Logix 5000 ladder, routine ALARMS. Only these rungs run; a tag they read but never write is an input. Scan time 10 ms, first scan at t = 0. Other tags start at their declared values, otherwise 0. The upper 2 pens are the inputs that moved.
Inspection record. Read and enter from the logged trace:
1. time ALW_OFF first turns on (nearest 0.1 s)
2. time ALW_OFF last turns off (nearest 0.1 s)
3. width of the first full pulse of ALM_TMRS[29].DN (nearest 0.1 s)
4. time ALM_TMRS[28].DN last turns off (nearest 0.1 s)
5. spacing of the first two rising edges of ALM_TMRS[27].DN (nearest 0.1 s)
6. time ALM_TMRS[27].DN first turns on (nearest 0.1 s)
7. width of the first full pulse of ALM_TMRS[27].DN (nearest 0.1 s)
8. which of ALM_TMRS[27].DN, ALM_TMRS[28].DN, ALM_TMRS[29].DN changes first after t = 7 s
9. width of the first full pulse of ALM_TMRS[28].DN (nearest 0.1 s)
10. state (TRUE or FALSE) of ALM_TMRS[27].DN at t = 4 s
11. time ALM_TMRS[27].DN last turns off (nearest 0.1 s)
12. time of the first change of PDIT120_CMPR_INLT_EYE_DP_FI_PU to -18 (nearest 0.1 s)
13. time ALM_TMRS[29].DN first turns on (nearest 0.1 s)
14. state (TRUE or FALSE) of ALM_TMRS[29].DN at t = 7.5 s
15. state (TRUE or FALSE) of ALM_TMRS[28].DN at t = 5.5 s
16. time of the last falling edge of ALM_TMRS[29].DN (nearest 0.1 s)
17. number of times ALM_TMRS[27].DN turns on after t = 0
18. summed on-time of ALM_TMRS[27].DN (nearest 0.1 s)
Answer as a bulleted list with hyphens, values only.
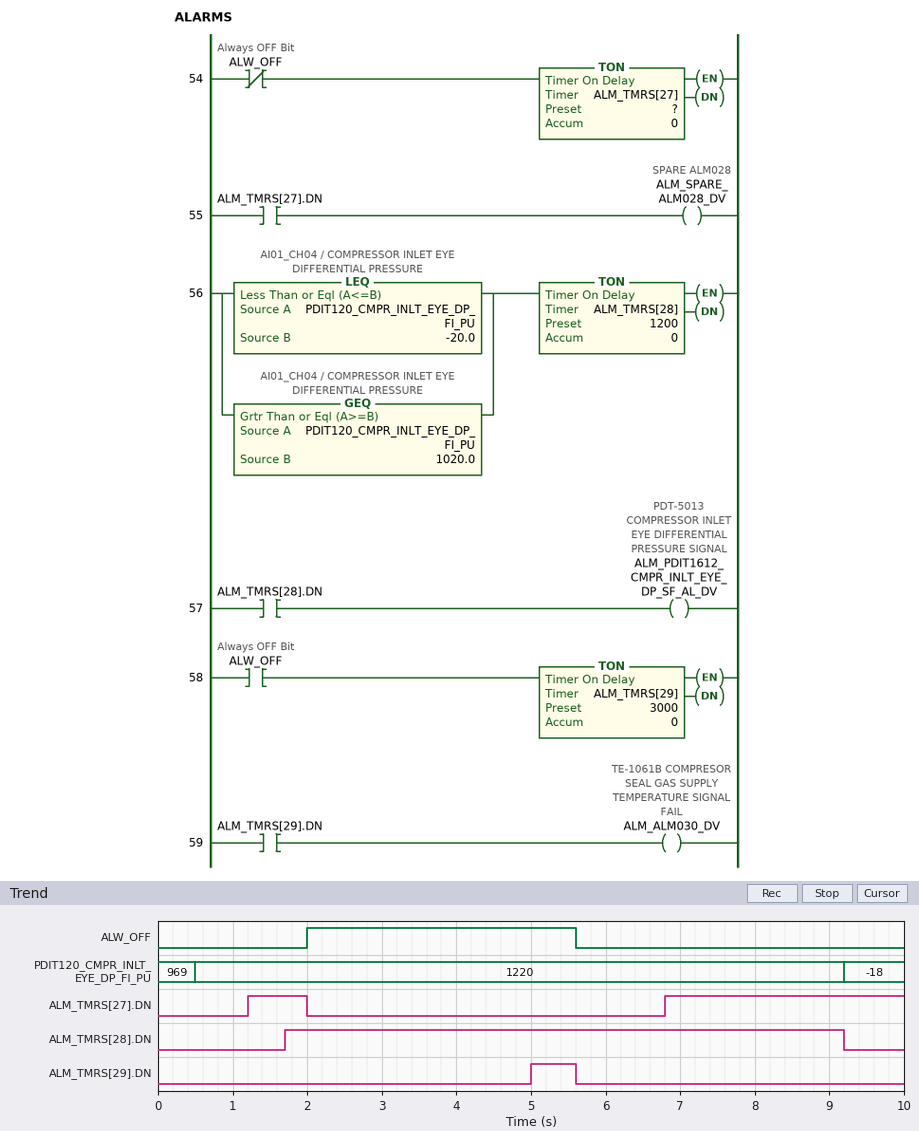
- 2.0 s
- 5.6 s
- 0.6 s
- 9.2 s
- 5.6 s
- 1.2 s
- 0.8 s
- ALM_TMRS[28].DN
- 7.5 s
- FALSE
- 2.0 s
- 9.2 s
- 5.0 s
- FALSE
- TRUE
- 5.6 s
- 2
- 4.0 s
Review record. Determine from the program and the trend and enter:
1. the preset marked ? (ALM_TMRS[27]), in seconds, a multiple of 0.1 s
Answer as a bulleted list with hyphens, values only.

- 1.2 s
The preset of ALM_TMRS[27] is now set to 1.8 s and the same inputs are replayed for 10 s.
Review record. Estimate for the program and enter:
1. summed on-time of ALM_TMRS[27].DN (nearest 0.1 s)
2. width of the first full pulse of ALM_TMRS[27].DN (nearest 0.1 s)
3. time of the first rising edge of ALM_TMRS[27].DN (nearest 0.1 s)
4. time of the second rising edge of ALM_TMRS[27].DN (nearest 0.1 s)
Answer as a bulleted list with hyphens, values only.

- 2.8 s
- 0.2 s
- 1.8 s
- 7.4 s
